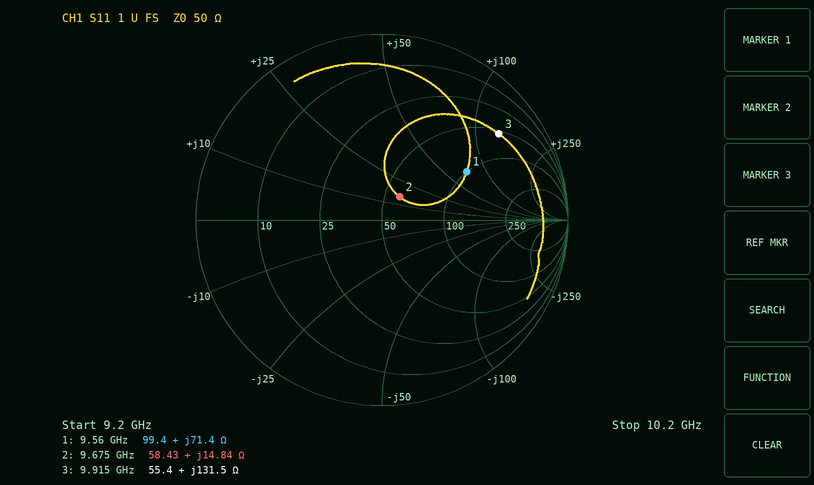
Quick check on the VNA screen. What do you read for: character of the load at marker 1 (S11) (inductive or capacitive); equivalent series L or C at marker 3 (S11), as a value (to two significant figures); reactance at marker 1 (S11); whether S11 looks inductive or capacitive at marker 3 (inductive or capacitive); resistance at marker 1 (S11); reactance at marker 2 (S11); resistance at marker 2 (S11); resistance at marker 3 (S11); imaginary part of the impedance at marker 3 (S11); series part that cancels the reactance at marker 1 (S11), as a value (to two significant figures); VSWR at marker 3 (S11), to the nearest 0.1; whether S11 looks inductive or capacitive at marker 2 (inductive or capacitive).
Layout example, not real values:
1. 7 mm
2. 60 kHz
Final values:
1. inductive
2. 2.1 nH
3. +71.4 Ω
4. inductive
5. 99.4 Ω
6. +14.84 Ω
7. 58.43 Ω
8. 55.4 Ω
9. +131.5 Ω
10. 230 fF
11. 8.1
12. inductive
